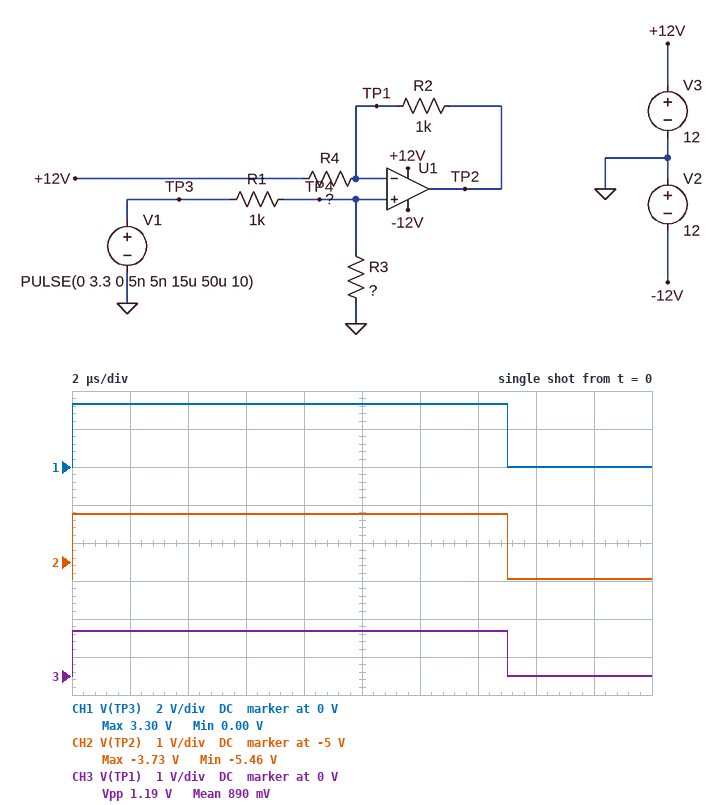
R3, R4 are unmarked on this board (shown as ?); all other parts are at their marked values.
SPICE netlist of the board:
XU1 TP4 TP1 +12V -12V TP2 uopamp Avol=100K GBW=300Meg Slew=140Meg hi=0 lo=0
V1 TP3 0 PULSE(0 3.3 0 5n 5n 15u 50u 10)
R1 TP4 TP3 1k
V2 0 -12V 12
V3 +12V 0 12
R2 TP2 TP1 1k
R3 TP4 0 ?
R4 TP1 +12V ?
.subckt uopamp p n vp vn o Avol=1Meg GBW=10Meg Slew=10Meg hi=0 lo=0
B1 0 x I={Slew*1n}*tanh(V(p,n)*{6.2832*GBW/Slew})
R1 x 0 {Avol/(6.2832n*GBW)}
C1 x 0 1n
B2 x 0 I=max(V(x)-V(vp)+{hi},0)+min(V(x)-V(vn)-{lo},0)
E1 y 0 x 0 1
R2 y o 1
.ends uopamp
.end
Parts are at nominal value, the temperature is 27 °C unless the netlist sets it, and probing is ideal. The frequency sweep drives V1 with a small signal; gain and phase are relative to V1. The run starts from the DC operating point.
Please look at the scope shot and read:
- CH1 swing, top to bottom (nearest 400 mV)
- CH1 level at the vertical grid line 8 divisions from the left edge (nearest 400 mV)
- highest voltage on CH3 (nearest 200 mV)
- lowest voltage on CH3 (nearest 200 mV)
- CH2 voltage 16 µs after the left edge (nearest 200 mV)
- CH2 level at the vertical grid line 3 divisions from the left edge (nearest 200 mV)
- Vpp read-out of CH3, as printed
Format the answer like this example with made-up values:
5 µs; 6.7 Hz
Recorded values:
3.2 V; 0 V; 1.2 V; 0 V; -5.4 V; -3.8 V; 1.19 V
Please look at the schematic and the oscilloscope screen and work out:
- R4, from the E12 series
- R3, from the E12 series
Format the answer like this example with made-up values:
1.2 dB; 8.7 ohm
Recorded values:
2.2 kΩ; 560 Ω
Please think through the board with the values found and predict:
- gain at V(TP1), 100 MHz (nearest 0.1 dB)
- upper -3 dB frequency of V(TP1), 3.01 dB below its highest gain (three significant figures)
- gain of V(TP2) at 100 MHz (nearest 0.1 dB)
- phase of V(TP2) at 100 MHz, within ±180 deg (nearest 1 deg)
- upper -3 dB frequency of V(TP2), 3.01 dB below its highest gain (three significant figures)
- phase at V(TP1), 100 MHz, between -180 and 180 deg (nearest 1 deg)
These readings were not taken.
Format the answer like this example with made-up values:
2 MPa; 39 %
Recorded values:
-9.8 dB; 206 MHz; -6.6 dB; -26 deg; 206 MHz; -26 deg
